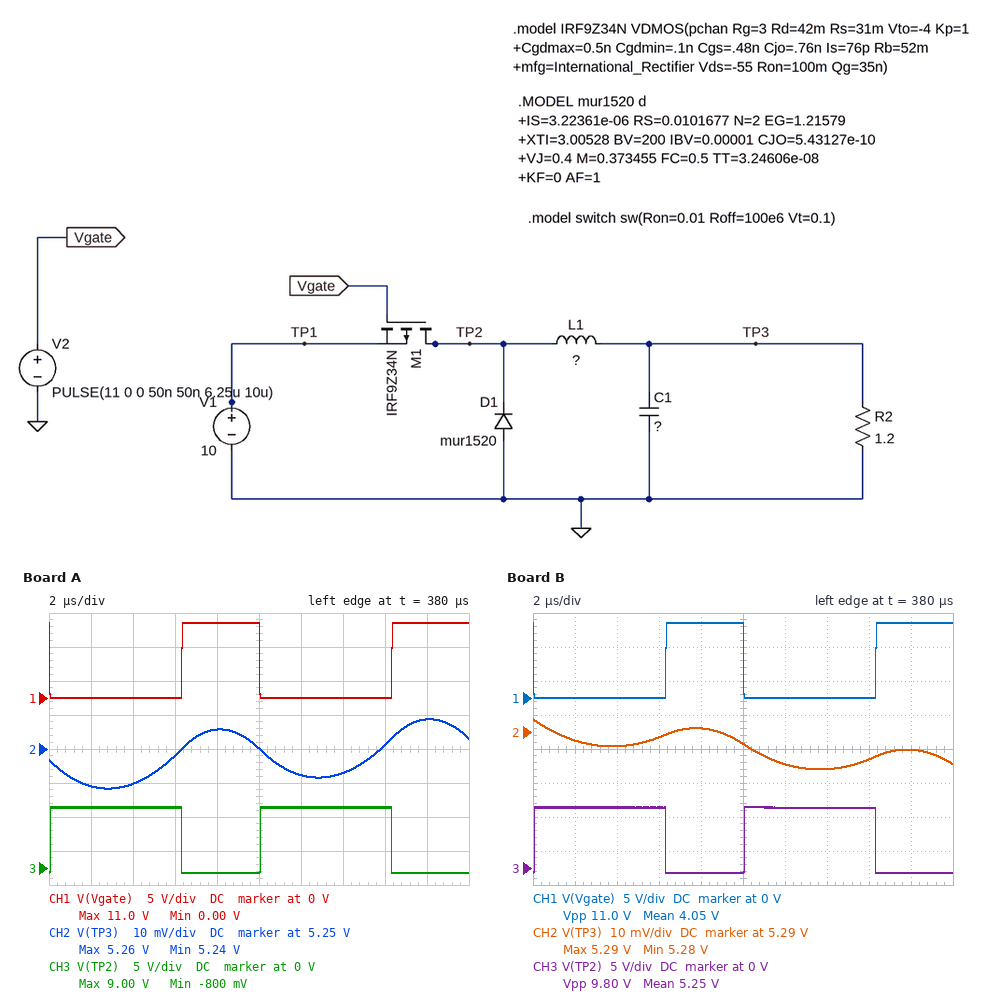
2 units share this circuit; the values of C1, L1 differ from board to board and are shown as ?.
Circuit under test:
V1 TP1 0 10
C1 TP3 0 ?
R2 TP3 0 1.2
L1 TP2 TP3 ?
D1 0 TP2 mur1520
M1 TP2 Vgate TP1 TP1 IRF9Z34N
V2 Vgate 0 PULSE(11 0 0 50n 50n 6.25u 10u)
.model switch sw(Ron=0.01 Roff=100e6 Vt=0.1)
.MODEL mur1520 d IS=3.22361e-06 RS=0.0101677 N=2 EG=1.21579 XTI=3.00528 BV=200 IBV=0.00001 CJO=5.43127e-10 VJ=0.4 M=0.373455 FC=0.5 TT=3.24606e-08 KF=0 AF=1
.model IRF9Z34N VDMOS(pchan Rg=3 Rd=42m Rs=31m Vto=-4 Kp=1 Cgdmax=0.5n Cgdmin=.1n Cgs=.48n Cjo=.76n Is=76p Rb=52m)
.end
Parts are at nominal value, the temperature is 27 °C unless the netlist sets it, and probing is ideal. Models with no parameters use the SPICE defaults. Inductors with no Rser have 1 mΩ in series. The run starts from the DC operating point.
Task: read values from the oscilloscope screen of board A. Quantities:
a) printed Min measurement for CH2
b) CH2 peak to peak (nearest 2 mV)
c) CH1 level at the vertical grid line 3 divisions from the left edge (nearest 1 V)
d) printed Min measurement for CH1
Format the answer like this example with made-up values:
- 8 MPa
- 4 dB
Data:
- 5.24 V
- 20 mV
- 0 V
- 0.00 V
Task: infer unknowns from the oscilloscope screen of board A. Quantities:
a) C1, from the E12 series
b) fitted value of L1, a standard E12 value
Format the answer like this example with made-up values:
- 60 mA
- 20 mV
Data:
- 15 µF
- 120 µH
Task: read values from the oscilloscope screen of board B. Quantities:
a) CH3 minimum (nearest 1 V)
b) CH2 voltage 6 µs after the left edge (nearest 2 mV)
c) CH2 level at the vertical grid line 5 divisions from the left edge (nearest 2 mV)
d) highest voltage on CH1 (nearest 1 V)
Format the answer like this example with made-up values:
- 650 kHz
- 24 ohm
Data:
- -1 V
- 5.288 V
- 5.286 V
- 11 V
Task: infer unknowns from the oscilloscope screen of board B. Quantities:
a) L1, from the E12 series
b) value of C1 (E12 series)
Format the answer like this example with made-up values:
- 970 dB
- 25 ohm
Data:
- 100 µH
- 33 µF
